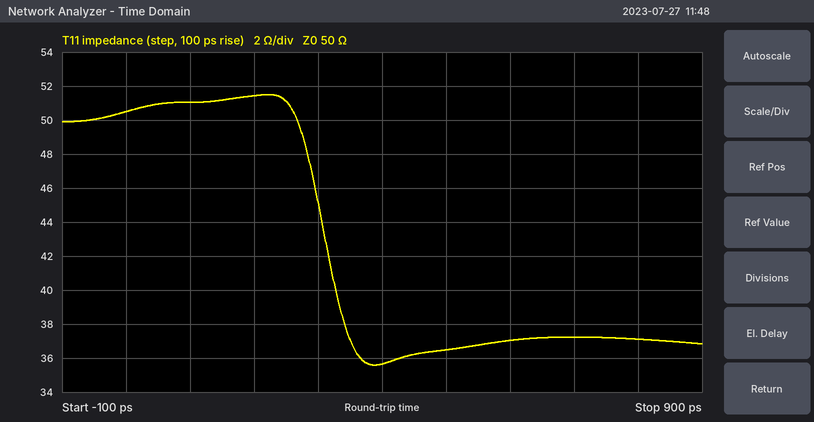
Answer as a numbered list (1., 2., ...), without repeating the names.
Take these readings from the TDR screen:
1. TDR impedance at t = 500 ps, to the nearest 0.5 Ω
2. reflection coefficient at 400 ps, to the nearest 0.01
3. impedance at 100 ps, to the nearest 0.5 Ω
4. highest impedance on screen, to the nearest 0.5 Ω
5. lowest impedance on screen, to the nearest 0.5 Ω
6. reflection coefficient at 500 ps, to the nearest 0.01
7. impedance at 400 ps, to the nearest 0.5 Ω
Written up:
1. 36.5 Ω
2. -0.17
3. 51.0 Ω
4. 51.5 Ω
5. 35.5 Ω
6. -0.16
7. 35.5 Ω
